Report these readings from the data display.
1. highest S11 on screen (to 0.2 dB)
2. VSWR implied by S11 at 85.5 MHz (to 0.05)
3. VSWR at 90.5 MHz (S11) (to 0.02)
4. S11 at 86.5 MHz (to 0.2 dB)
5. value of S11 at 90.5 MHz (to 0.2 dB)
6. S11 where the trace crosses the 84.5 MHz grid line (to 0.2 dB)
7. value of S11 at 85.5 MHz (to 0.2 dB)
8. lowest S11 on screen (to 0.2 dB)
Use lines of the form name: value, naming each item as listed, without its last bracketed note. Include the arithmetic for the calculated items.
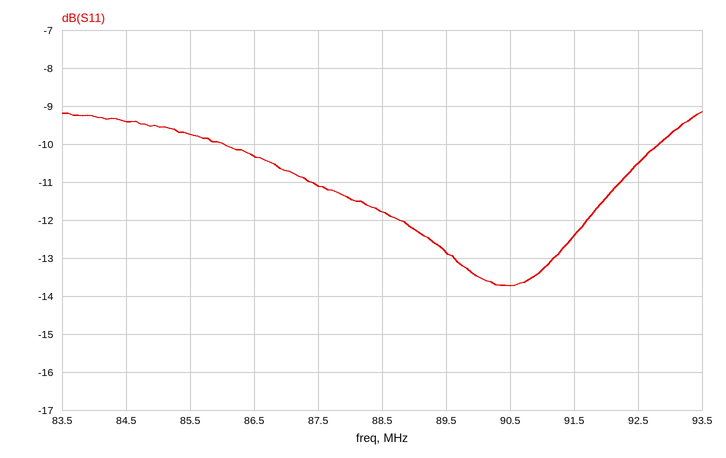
highest S11 on screen: -9.2 dB
VSWR implied by S11 at 85.5 MHz: |Γ| = 10^(-9.8/20) = 0.3236; VSWR = (1 + 0.3236)/(1 − 0.3236) ≈ 1.96, so 1.95 to the nearest 0.05
VSWR at 90.5 MHz (S11): |Γ| = 10^(-13.8/20) = 0.2042; VSWR = (1 + 0.2042)/(1 − 0.2042) ≈ 1.51, so 1.52 to the nearest 0.02
S11 at 86.5 MHz: -10.4 dB
value of S11 at 90.5 MHz: -13.8 dB
S11 where the trace crosses the 84.5 MHz grid line: -9.4 dB
value of S11 at 85.5 MHz: -9.8 dB
lowest S11 on screen: -13.8 dB
